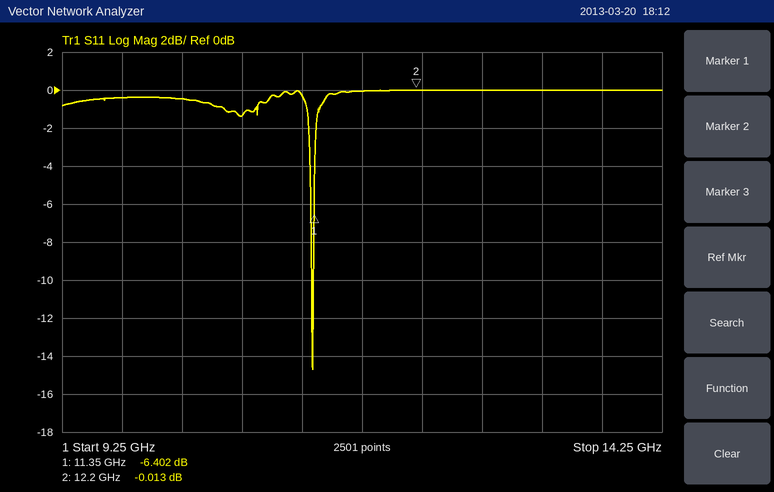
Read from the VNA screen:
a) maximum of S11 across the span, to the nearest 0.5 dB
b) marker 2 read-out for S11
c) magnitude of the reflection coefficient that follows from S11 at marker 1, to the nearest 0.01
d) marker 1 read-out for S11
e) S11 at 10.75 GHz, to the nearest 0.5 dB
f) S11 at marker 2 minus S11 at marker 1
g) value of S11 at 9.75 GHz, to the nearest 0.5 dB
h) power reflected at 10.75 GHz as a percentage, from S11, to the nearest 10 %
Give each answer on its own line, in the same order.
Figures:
0.0 dB
-0.013 dB
0.48
-6.402 dB
-1.5 dB
6.389 dB
-0.5 dB
70 %
